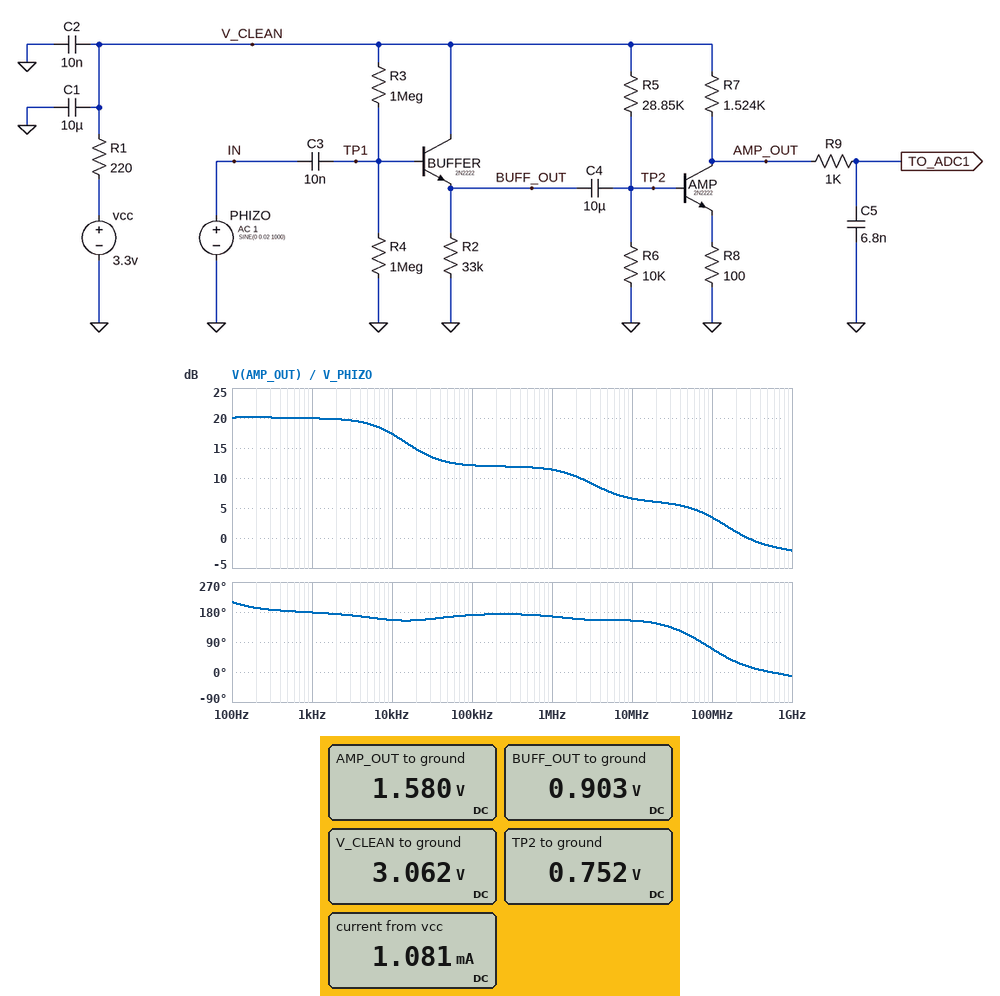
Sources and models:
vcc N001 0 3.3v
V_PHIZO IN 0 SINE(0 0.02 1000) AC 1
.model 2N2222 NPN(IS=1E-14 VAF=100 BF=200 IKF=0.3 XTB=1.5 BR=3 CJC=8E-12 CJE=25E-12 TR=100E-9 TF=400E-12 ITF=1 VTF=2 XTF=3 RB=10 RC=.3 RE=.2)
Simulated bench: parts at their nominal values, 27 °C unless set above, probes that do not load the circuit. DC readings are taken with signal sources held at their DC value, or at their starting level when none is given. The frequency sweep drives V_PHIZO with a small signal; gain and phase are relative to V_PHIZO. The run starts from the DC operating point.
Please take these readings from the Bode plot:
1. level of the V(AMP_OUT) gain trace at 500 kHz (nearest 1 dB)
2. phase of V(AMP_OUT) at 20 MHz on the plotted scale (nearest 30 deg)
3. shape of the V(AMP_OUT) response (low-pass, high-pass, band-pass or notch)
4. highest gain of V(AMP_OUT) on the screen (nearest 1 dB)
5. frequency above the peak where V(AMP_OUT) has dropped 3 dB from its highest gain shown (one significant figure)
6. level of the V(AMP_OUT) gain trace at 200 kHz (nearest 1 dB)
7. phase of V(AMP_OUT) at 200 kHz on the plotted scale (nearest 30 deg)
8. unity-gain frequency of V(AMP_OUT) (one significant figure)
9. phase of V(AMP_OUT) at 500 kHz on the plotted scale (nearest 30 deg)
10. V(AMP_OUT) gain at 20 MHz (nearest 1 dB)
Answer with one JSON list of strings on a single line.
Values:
["12 dB", "150 deg", "low-pass", "20 dB", "10 kHz", "12 dB", "180 deg", "300 MHz", "180 deg", "6 dB"]
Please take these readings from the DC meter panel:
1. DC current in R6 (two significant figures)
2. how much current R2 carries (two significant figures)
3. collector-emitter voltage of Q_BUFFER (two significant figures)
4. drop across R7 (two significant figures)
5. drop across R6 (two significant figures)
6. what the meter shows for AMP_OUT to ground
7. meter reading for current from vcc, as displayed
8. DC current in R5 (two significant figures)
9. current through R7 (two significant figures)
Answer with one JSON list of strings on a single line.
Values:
["75 µA", "27 µA", "2.2 V", "1.5 V", "750 mV", "1.580 V", "1.081 mA", "80 µA", "970 µA"]
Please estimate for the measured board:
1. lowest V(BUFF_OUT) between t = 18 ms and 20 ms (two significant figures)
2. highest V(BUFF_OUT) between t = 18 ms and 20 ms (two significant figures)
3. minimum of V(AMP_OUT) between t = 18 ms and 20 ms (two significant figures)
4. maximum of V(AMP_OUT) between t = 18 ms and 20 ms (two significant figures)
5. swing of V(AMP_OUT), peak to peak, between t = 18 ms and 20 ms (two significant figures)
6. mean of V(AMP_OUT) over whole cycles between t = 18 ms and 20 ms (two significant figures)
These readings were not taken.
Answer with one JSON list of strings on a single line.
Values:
["890 mV", "920 mV", "1.4 V", "1.8 V", "400 mV", "1.6 V"]
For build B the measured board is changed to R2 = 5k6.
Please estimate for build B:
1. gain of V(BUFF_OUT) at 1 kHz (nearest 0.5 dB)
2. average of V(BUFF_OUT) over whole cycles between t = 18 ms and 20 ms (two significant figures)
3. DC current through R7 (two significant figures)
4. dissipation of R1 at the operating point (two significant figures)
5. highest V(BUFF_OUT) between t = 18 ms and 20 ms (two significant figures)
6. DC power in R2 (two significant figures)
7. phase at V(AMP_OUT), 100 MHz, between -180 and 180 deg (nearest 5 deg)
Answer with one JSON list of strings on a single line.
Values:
["-0.5 dB", "640 mV", "950 µA", "290 µW", "660 mV", "74 µW", "65 deg"]
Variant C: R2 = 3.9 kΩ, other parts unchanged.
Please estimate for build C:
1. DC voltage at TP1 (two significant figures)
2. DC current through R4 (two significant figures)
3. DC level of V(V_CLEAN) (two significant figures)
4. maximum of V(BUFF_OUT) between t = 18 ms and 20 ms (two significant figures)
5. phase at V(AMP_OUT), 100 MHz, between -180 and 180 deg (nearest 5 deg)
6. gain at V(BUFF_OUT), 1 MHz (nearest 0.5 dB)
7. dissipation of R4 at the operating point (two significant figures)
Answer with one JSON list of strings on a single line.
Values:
["1.2 V", "1.2 µA", "3.0 V", "580 mV", "65 deg", "-0.5 dB", "1.4 µW"]
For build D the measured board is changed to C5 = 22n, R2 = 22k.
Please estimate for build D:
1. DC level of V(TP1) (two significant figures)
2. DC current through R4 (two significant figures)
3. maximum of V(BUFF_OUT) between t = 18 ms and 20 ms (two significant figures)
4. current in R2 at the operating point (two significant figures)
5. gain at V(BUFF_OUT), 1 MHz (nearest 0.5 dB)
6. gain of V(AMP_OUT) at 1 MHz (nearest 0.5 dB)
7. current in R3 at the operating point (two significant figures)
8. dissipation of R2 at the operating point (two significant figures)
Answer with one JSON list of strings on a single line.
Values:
["1.4 V", "1.4 µA", "880 mV", "39 µA", "-1.5 dB", "12.0 dB", "1.6 µA", "34 µW"]
